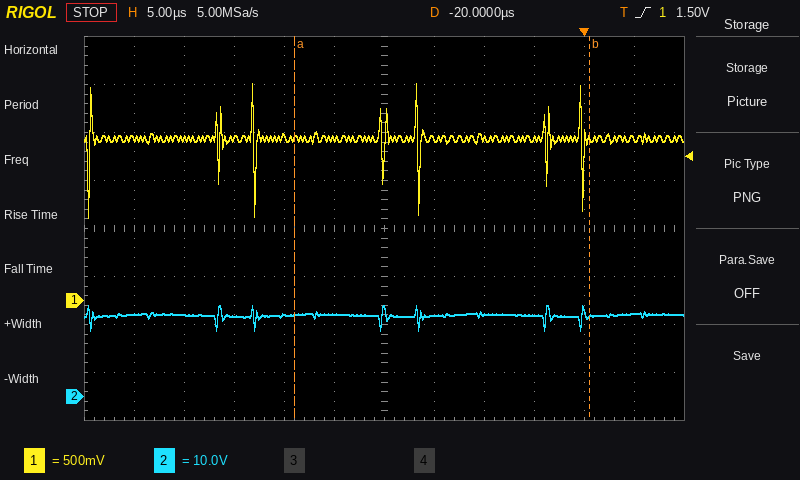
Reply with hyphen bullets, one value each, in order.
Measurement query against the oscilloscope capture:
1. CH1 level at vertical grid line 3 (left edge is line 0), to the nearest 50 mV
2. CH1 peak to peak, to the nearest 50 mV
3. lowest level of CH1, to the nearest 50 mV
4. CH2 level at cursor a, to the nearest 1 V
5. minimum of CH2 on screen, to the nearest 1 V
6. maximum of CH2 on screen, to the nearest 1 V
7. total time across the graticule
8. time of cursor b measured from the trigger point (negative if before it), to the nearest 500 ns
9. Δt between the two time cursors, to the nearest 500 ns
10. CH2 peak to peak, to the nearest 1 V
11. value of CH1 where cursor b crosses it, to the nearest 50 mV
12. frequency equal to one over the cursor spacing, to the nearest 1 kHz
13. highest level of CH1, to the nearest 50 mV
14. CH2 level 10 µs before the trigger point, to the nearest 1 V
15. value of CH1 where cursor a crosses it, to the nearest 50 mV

- 1.70 V
- 1.40 V
- 850 mV
- 17 V
- 14 V
- 19 V
- 60 µs
- +500 ns
- 29.5 µs
- 5 V
- 1.65 V
- 34 kHz
- 2.25 V
- 17 V
- 1.70 V
